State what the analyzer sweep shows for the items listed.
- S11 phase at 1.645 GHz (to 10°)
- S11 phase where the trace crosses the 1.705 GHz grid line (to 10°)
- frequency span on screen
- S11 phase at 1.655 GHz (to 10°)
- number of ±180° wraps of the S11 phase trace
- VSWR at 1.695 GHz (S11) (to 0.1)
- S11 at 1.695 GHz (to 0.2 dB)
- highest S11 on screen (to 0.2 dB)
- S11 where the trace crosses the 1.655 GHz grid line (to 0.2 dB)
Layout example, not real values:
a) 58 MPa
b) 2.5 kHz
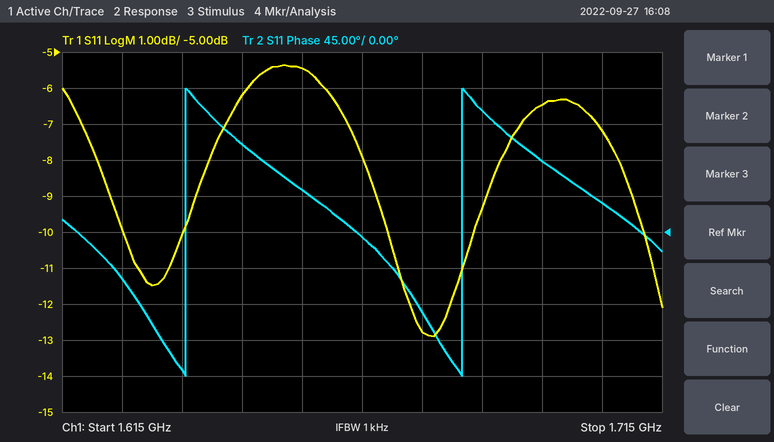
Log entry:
a) 110°
b) 40°
c) 100 MHz
d) 50°
e) 2
f) 2.8
g) -6.4 dB
h) -5.4 dB
i) -5.4 dB
